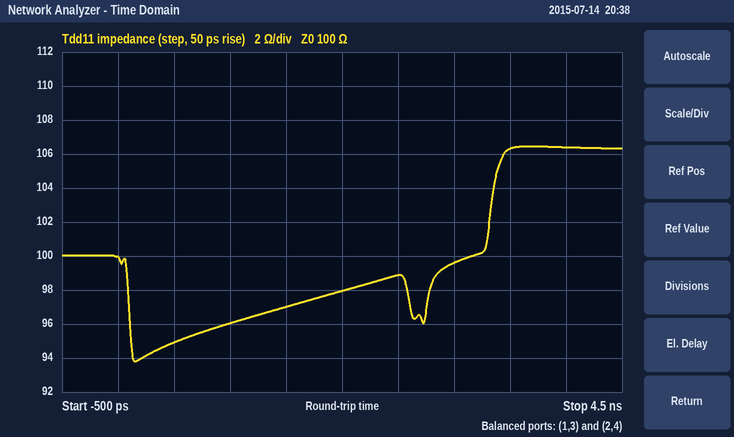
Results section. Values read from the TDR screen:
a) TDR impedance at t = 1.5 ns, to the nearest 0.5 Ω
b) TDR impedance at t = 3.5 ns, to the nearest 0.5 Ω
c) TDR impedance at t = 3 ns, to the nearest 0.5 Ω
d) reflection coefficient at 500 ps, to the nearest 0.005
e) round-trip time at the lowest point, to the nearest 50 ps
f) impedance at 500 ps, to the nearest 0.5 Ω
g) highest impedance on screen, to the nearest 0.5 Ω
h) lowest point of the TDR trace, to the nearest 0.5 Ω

97.0 Ω
106.5 Ω
99.5 Ω
-0.025
150 ps
95.0 Ω
106.5 Ω
94.0 Ω
